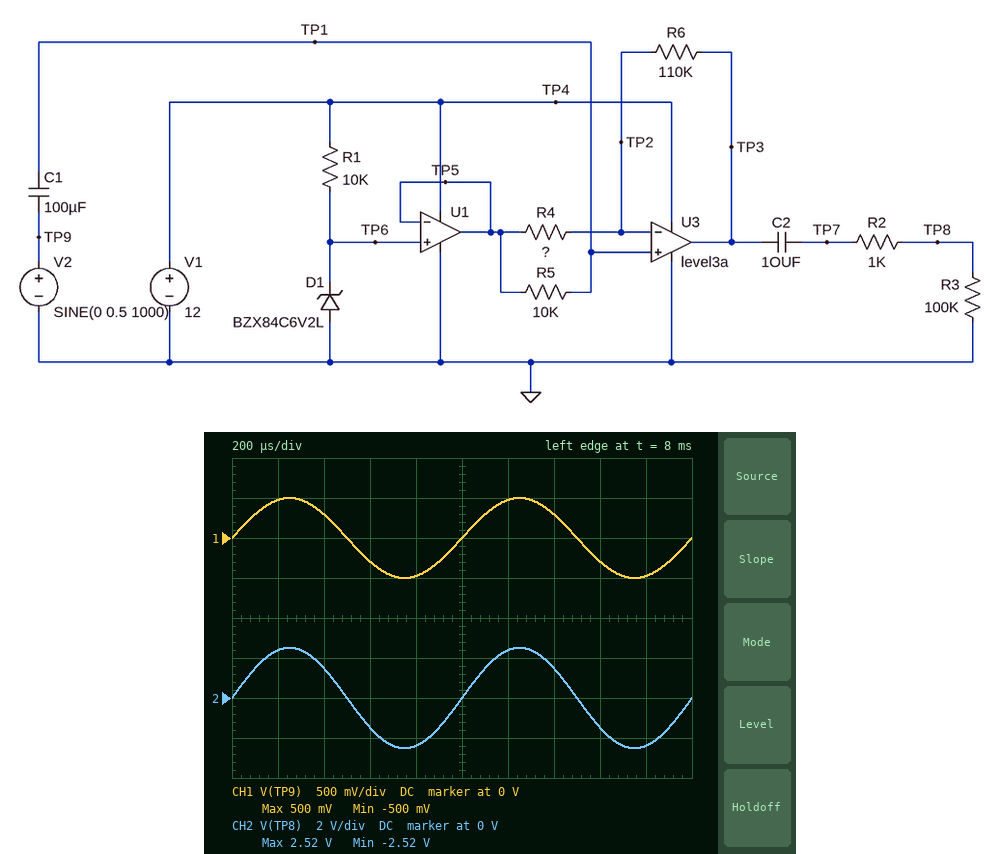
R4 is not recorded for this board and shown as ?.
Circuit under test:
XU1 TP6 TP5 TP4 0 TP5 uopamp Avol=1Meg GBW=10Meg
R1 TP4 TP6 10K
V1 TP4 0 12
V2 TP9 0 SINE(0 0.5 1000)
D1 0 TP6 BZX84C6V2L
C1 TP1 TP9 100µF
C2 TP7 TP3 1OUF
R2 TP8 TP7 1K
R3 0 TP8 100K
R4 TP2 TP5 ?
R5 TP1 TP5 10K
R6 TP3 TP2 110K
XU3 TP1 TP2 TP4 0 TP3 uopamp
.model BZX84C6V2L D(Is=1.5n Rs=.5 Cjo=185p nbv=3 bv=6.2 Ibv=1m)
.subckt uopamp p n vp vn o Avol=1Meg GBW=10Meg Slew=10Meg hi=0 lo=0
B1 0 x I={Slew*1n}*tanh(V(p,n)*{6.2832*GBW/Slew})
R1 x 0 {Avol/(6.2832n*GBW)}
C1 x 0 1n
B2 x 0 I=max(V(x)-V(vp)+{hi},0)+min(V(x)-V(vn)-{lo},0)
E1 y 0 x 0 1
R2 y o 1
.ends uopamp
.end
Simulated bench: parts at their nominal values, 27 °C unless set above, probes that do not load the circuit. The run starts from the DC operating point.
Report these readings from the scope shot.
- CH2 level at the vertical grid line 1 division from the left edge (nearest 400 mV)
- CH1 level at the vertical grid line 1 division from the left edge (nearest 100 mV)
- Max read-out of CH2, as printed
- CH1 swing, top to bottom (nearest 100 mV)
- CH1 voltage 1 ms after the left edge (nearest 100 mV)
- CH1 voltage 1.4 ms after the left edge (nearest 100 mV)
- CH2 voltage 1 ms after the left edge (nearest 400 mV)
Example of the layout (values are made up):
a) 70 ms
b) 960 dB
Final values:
a) 2.4 V
b) 500 mV
c) 2.52 V
d) 1.0 V
e) 0 V
f) 300 mV
g) 0 V
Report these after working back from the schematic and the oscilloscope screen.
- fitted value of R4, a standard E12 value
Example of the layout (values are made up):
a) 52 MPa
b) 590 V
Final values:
a) 27 kΩ
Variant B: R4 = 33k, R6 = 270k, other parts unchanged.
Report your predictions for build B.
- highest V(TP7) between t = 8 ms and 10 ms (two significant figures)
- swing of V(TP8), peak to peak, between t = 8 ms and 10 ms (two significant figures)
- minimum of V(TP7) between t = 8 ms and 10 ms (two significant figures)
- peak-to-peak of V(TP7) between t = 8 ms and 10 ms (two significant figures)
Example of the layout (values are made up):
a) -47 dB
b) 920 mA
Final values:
a) 4.6 V
b) 9.1 V
c) -4.6 V
d) 9.2 V
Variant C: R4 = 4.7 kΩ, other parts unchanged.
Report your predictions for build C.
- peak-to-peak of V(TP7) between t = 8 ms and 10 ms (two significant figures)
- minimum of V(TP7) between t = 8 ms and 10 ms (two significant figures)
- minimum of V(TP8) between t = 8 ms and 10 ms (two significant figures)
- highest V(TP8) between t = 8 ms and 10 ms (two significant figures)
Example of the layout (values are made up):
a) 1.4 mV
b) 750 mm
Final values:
a) 12 V
b) -6.2 V
c) -6.1 V
d) 5.8 V
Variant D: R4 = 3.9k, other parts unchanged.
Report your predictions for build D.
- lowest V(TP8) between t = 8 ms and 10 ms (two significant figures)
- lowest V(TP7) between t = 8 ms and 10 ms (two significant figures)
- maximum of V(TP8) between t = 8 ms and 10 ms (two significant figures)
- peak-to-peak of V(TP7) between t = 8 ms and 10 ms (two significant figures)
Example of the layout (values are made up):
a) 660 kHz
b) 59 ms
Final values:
a) -6.1 V
b) -6.2 V
c) 5.8 V
d) 12 V
